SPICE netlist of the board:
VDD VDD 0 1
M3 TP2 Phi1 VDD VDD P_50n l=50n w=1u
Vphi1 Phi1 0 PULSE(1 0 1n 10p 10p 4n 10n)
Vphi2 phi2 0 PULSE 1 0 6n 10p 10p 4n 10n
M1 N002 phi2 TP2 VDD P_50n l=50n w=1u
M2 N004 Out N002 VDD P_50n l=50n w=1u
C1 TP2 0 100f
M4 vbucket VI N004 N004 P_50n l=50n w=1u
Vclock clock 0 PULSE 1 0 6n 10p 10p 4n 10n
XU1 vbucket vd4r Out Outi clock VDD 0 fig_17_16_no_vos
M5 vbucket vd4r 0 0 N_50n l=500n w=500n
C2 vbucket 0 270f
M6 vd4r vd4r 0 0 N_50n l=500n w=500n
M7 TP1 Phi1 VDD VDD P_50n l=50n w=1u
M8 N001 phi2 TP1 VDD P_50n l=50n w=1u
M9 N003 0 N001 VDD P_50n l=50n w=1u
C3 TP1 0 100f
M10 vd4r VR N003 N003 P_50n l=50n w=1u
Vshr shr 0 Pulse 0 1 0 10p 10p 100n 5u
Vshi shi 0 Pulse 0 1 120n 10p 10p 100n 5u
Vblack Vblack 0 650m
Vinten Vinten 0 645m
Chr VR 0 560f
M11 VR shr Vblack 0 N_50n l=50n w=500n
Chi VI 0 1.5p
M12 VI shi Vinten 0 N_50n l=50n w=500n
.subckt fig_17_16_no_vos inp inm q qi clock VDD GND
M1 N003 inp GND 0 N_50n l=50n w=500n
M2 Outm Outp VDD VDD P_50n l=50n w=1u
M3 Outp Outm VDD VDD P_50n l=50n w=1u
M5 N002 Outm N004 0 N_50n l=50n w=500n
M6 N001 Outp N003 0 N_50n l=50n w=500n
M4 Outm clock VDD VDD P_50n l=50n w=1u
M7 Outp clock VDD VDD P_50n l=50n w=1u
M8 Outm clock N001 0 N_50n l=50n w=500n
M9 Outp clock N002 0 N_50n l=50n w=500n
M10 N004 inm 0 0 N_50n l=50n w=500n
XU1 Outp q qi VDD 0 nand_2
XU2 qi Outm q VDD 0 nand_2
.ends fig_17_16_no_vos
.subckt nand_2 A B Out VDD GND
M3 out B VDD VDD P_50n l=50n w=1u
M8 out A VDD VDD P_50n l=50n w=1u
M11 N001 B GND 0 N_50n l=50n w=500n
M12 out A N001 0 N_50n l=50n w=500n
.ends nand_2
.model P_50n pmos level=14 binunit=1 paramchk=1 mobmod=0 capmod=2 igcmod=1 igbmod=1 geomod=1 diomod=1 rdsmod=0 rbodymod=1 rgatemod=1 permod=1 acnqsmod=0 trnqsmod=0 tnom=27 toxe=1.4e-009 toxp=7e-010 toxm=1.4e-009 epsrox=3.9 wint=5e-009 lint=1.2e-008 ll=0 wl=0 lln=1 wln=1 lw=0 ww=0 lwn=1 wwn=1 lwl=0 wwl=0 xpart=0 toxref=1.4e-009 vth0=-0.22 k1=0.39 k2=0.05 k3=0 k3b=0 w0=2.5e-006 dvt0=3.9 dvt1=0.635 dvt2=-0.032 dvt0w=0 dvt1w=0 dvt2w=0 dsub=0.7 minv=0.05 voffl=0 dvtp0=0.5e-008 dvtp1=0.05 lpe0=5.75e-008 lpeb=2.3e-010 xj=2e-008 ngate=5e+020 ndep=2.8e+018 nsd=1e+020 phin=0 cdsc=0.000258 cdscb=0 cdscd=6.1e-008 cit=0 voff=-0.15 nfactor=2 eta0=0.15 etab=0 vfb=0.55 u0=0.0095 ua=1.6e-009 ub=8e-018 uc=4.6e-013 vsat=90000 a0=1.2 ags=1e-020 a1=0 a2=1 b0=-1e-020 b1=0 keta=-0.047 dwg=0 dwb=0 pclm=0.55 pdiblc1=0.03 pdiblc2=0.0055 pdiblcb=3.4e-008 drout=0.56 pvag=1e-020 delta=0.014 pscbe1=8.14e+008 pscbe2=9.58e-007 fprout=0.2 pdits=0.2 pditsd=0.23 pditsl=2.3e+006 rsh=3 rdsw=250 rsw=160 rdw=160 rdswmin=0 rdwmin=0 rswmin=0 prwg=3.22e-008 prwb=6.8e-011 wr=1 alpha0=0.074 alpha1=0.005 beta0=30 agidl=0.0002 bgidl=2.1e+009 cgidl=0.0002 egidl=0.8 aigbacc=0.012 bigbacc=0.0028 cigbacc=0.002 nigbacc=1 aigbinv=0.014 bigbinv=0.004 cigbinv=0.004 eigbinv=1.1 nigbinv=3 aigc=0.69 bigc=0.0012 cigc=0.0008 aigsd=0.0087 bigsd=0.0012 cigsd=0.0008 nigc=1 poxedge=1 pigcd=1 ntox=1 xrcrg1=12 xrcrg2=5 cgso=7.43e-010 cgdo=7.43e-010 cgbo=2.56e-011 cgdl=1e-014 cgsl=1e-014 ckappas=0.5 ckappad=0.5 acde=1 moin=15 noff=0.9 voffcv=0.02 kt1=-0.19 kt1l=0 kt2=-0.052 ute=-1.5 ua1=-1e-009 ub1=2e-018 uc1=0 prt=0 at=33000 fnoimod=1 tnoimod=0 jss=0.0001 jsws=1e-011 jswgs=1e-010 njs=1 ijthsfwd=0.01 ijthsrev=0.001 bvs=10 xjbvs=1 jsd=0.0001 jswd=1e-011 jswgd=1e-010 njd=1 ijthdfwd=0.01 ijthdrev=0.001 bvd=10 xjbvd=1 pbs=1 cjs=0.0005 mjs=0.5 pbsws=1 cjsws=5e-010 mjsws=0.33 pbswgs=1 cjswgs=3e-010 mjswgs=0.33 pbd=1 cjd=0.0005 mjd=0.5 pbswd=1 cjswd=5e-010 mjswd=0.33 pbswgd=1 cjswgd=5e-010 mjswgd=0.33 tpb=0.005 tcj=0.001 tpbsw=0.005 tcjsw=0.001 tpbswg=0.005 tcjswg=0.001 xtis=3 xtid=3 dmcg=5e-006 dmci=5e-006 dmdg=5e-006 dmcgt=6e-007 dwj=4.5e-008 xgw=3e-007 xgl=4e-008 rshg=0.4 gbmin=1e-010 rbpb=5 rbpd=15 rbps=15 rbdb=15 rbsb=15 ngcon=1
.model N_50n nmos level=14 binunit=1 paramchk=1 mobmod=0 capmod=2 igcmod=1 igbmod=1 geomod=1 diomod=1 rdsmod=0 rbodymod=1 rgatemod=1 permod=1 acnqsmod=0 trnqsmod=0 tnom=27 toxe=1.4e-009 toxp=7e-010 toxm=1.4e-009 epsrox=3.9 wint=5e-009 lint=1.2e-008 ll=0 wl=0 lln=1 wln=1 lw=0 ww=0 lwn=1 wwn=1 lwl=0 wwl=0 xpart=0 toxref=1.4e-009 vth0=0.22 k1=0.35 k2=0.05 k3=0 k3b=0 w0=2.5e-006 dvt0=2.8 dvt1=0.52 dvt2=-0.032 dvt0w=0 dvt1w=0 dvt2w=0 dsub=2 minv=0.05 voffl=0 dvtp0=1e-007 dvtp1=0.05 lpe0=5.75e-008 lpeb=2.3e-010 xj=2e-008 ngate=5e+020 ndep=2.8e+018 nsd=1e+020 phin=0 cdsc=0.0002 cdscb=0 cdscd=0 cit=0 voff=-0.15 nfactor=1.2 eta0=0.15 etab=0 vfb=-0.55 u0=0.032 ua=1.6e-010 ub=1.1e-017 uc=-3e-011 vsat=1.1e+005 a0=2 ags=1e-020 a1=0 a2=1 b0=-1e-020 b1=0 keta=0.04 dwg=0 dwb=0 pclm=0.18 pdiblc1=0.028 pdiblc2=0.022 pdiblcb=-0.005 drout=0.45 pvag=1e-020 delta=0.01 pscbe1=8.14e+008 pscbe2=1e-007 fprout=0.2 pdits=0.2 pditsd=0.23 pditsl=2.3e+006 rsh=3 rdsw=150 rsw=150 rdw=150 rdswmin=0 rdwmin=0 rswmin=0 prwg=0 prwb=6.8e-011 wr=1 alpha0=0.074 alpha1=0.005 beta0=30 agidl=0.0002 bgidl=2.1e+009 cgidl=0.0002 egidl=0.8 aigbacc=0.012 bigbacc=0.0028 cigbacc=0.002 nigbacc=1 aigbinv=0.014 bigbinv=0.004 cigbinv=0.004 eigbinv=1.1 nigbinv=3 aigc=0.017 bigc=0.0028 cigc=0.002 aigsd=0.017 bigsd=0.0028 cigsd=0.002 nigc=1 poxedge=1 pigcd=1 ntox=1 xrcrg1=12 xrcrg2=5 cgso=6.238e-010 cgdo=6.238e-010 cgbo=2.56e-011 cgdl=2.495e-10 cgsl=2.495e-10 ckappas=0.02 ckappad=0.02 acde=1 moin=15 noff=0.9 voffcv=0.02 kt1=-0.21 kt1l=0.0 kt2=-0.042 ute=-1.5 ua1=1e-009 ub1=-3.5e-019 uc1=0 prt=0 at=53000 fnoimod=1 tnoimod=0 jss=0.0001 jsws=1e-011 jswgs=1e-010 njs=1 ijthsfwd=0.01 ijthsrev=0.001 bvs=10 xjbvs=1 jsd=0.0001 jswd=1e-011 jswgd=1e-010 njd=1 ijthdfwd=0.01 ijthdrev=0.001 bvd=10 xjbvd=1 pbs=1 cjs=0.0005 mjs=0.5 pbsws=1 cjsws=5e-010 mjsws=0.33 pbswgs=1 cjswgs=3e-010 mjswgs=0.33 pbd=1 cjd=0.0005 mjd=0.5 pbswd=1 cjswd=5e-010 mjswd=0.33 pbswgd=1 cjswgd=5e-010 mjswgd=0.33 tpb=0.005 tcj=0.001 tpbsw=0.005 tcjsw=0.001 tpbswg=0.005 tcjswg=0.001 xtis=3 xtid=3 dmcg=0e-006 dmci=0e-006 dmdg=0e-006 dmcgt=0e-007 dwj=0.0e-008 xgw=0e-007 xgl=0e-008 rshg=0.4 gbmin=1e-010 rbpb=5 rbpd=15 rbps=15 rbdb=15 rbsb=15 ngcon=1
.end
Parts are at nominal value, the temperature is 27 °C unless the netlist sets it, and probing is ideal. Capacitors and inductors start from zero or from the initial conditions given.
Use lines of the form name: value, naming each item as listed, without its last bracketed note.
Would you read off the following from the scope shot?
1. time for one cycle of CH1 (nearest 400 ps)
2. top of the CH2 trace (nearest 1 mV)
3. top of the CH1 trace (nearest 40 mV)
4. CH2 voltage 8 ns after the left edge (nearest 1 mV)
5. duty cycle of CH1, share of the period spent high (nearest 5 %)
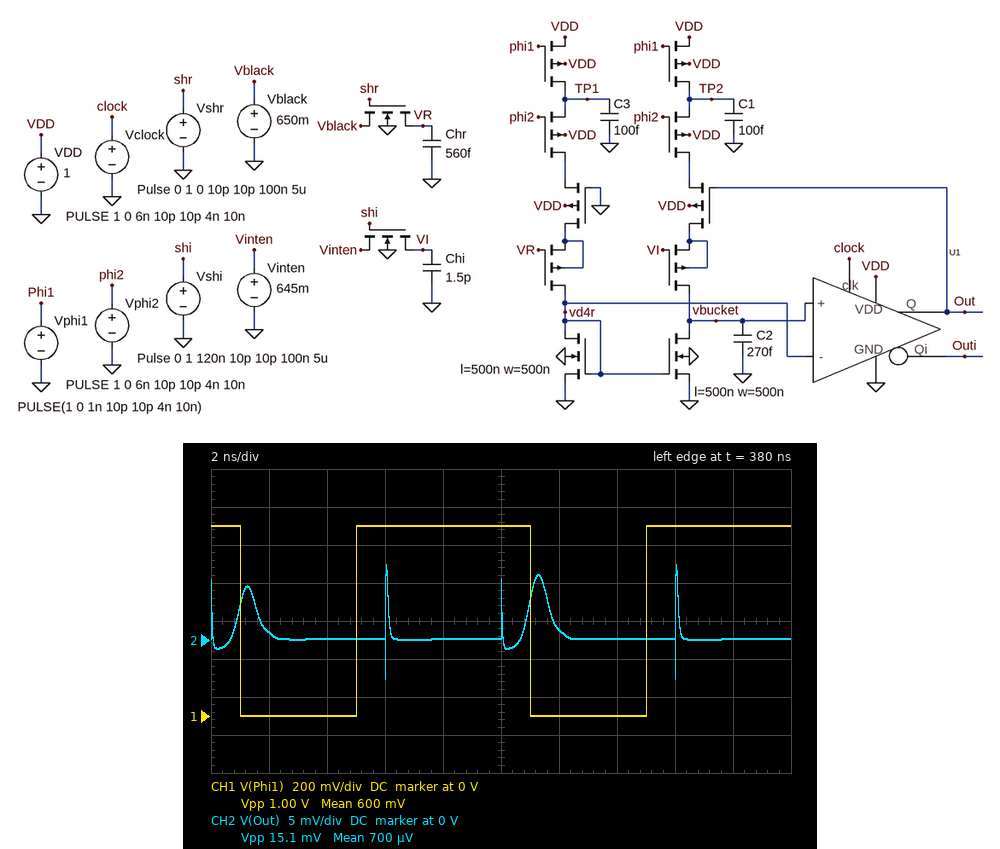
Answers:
time for one cycle of CH1: 10.0 ns
top of the CH2 trace: 10 mV
top of the CH1 trace: 1.00 V
CH2 voltage 8 ns after the left edge: 0 V
duty cycle of CH1, share of the period spent high: 60 %
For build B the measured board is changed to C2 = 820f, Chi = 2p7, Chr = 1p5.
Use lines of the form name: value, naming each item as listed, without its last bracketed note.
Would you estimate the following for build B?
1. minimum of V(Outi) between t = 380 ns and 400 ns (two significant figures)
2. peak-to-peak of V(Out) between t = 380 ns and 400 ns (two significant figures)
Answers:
minimum of V(Outi) between t = 380 ns and 400 ns: -6.3 mV
peak-to-peak of V(Out) between t = 380 ns and 400 ns: 1.0 V
